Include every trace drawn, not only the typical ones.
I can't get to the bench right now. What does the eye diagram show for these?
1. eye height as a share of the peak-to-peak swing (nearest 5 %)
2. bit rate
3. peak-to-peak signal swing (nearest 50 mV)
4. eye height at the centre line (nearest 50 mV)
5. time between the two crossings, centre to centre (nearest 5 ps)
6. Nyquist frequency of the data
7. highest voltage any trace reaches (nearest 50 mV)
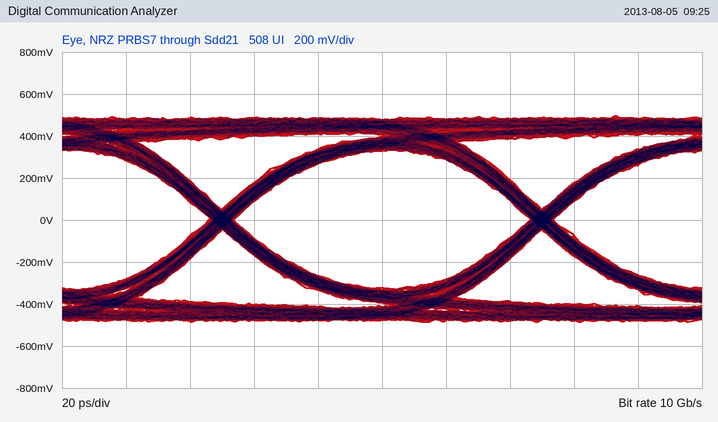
65 %
10 Gb/s
1.00 V
650 mV
100 ps
5 GHz
500 mV
